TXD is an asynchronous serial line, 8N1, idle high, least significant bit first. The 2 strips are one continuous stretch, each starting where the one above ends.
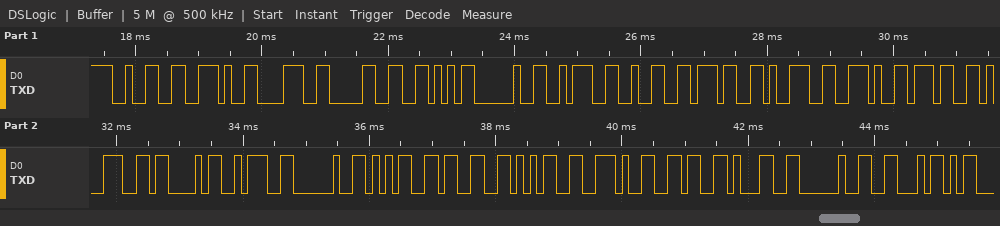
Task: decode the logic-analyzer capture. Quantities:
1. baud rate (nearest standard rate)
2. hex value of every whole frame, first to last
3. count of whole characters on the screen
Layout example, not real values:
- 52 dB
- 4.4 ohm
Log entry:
- 9600 baud
- 32 2E 38 30 56 20 3A 32 37 39 2E 37 39 43 3A 20 35 33 35 2E 36 31 20 46
- 24
